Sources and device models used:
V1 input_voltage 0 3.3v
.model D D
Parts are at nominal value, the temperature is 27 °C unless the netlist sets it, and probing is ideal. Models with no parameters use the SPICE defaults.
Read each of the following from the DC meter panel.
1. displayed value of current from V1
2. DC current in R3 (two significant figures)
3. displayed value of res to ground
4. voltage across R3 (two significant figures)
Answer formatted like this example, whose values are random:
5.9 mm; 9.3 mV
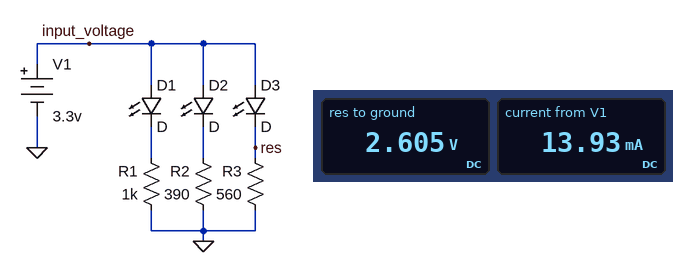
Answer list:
13.93 mA; 4.7 mA; 2.605 V; 2.6 V
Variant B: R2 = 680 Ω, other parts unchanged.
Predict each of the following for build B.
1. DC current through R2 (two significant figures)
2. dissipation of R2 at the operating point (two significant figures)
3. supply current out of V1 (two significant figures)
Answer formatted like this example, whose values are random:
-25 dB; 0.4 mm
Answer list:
3.8 mA; 10 mW; 11 mA
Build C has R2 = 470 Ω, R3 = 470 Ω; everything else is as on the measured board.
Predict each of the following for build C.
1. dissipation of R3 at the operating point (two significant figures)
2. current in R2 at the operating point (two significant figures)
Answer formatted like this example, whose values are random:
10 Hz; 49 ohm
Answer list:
14 mW; 5.5 mA
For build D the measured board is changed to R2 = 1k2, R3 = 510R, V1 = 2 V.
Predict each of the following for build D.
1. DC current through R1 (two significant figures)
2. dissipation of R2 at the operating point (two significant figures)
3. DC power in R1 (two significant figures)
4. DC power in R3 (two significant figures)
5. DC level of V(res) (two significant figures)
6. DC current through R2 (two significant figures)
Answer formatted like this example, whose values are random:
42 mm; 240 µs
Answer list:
1.3 mA; 1.5 mW; 1.8 mW; 3.4 mW; 1.3 V; 1.1 mA
